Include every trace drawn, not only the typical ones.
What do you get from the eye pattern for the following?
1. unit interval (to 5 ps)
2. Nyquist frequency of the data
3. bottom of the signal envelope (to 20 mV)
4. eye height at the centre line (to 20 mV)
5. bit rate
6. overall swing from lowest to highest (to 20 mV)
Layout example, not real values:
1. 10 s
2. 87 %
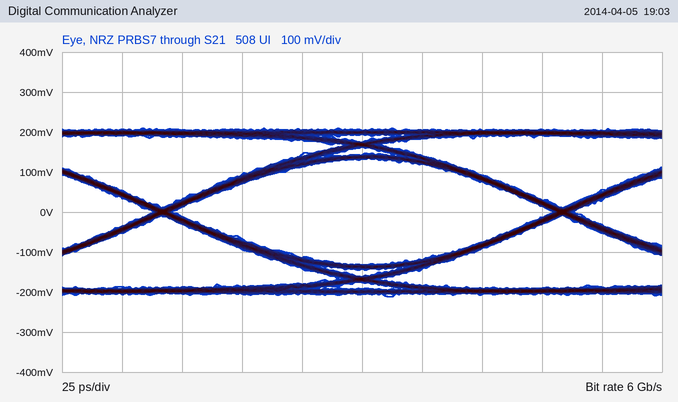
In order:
1. 165 ps
2. 3 GHz
3. -220 mV
4. 260 mV
5. 6 Gb/s
6. 420 mV
